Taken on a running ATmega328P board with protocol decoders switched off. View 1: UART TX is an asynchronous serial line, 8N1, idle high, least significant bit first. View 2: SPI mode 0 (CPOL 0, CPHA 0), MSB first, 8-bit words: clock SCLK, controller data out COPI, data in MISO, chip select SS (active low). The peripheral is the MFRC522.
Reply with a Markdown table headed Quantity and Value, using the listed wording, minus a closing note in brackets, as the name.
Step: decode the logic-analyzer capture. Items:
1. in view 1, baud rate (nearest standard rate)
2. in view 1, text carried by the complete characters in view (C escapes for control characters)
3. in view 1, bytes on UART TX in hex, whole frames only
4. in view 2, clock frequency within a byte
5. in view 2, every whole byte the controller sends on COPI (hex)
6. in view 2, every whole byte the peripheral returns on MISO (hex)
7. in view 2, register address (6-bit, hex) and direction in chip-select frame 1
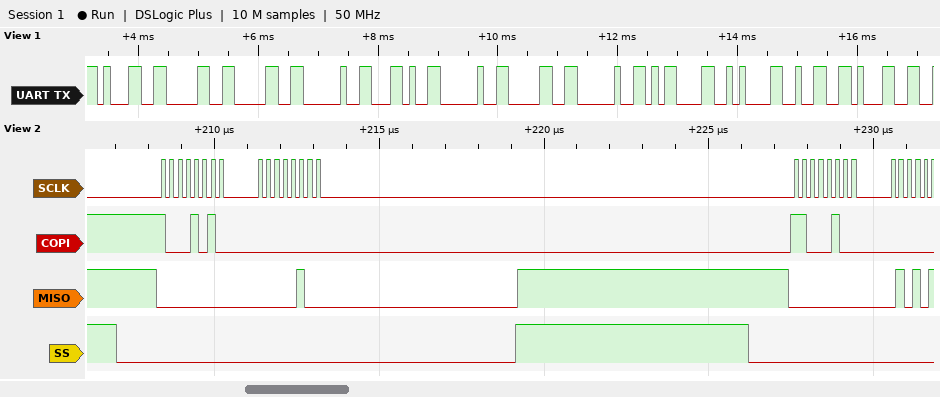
| Quantity | Value |
|---|---|
| in view 1, baud rate | 9600 baud |
| in view 1, text carried by the complete characters in view | "100 , 0 \r\n21" |
| in view 1, bytes on UART TX in hex, whole frames only | 31 30 30 20 2C 20 30 20 0D 0A 32 31 |
| in view 2, clock frequency within a byte | 4 MHz |
| in view 2, every whole byte the controller sends on COPI | 8A 00 C4 |
| in view 2, every whole byte the peripheral returns on MISO | 00 04 00 |
| in view 2, register address (6-bit, hex) and direction in chip-select frame 1 | 0x05 read |
